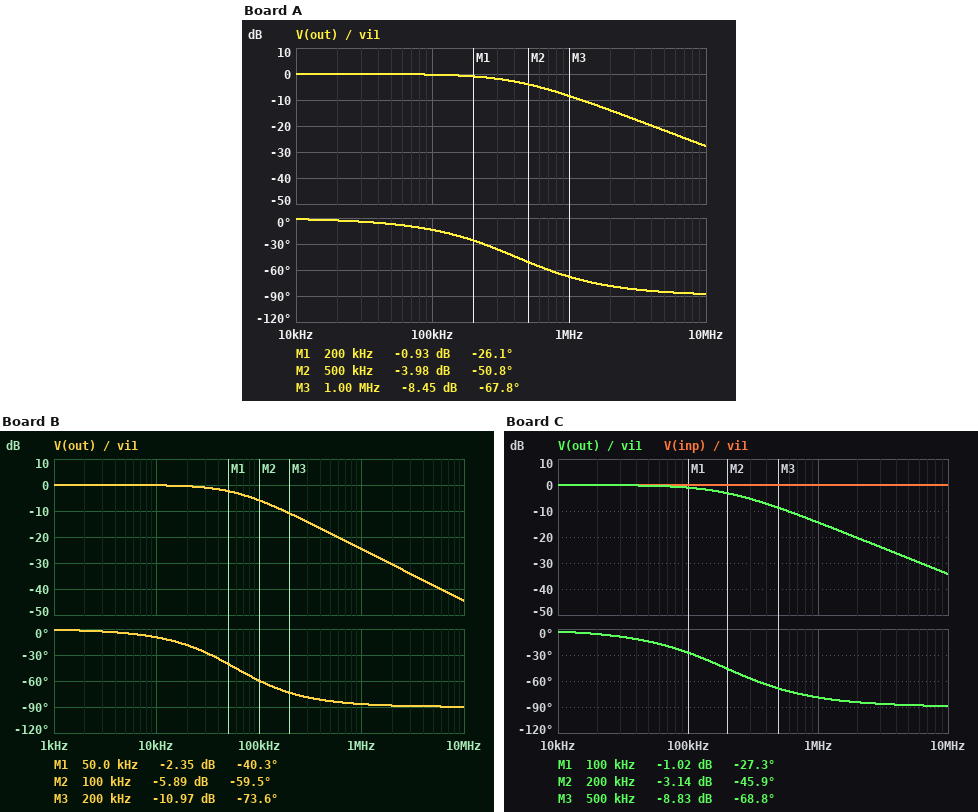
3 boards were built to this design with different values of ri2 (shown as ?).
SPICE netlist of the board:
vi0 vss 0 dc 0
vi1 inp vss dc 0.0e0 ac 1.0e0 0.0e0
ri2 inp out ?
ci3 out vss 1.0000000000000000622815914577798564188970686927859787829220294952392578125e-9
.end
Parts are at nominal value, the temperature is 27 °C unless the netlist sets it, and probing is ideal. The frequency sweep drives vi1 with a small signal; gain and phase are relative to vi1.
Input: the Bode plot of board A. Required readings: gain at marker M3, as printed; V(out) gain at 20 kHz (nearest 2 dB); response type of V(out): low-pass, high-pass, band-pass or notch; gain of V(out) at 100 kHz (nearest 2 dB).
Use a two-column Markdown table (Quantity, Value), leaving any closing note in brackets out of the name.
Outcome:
| Quantity | Value |
|---|---|
| gain at marker M3, as printed | -8.45 dB |
| V(out) gain at 20 kHz | 0 dB |
| response type of V(out): low-pass, high-pass, band-pass or notch | low-pass |
| gain of V(out) at 100 kHz | 0 dB |
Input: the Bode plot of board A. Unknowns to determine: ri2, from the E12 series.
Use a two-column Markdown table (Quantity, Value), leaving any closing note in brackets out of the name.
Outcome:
| Quantity | Value |
|---|---|
| ri2, from the E12 series | 390 Ω |
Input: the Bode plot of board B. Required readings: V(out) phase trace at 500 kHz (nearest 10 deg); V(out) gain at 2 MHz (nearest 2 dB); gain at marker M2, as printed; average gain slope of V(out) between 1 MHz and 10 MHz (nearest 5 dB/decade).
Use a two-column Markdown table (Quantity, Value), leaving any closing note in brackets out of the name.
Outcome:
| Quantity | Value |
|---|---|
| V(out) phase trace at 500 kHz | -80 deg |
| V(out) gain at 2 MHz | -30 dB |
| gain at marker M2, as printed | -5.89 dB |
| average gain slope of V(out) between 1 MHz and 10 MHz | -20 dB/decade |
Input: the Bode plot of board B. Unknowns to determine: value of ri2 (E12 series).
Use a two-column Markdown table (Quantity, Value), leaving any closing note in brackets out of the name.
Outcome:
| Quantity | Value |
|---|---|
| value of ri2 | 2.7 kΩ |
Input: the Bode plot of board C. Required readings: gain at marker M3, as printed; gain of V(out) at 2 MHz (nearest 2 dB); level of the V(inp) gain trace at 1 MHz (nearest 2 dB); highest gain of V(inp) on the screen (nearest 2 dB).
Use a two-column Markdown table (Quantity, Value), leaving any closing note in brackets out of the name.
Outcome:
| Quantity | Value |
|---|---|
| gain at marker M3, as printed | -8.83 dB |
| gain of V(out) at 2 MHz | -20 dB |
| level of the V(inp) gain trace at 1 MHz | 0 dB |
| highest gain of V(inp) on the screen | 0 dB |
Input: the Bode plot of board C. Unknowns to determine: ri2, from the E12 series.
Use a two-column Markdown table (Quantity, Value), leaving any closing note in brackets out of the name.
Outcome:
| Quantity | Value |
|---|---|
| ri2, from the E12 series | 820 Ω |
